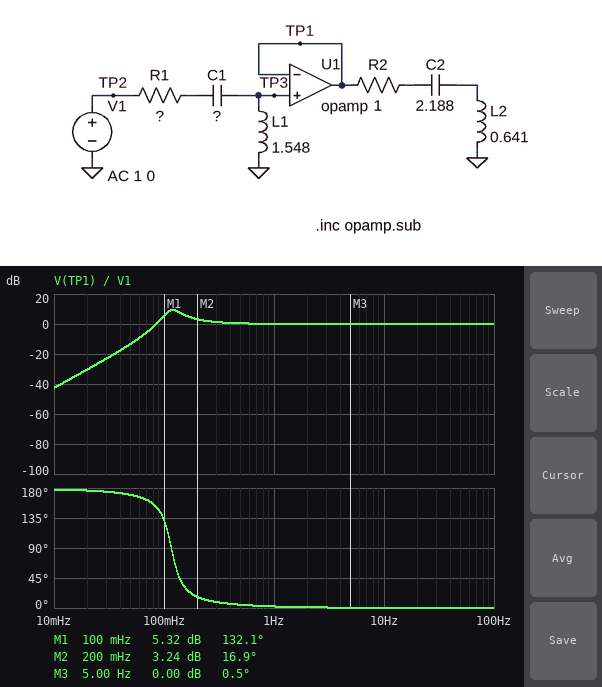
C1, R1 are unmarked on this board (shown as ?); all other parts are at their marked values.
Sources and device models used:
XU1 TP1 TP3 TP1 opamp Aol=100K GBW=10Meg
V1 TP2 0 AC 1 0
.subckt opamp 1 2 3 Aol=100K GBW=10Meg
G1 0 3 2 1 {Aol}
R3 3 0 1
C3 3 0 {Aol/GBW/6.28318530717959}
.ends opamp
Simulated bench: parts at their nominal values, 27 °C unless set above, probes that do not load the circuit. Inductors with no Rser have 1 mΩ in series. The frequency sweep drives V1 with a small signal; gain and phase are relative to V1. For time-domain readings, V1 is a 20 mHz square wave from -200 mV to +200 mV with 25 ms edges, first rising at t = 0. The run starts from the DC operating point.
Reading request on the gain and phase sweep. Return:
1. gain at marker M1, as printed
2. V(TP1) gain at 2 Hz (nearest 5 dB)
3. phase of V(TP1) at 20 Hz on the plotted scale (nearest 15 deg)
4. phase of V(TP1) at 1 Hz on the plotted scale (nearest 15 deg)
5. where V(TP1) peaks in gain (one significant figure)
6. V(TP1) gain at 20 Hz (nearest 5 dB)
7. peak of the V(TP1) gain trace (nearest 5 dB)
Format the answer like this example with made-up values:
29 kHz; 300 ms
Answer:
5.32 dB; 0 dB; 0 deg; 0 deg; 100 mHz; 0 dB; 10 dB
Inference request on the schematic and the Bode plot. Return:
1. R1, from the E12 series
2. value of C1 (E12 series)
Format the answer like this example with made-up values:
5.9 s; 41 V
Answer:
0.39 Ω; 1.2 F
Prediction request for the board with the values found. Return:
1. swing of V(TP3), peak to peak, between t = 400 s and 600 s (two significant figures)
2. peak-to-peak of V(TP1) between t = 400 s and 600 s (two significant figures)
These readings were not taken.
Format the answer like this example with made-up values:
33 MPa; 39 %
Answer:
770 mV; 770 mV
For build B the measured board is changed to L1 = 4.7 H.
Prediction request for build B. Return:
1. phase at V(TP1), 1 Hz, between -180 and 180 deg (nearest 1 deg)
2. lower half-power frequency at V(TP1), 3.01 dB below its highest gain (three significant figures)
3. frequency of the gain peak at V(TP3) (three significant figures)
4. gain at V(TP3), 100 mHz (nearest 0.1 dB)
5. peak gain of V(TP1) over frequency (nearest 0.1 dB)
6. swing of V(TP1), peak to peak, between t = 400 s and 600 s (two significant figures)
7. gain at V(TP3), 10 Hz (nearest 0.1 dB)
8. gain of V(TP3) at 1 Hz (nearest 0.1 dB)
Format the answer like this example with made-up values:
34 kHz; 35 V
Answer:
1 deg; 61.8 mHz; 67.7 mHz; 4.9 dB; 14.1 dB; 820 mV; 0 dB; 0 dB
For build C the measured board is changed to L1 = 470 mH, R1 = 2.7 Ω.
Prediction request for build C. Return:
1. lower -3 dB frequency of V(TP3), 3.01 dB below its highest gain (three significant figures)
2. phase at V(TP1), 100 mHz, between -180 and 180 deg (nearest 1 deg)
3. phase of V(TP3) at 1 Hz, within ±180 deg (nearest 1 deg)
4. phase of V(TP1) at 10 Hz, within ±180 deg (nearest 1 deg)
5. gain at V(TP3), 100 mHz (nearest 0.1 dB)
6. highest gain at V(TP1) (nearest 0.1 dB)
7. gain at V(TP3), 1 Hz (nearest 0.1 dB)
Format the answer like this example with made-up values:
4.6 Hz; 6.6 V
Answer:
866 mHz; 111 deg; 44 deg; 5 deg; -19.8 dB; 0 dB; -2.4 dB
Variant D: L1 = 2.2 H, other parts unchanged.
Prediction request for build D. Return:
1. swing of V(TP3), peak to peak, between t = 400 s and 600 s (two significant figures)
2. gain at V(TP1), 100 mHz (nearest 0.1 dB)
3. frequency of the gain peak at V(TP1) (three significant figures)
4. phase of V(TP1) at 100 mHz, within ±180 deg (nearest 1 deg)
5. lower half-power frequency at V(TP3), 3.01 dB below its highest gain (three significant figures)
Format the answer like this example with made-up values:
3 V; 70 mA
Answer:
890 mV; 10.9 dB; 100 mHz; 82 deg; 87.8 mHz
